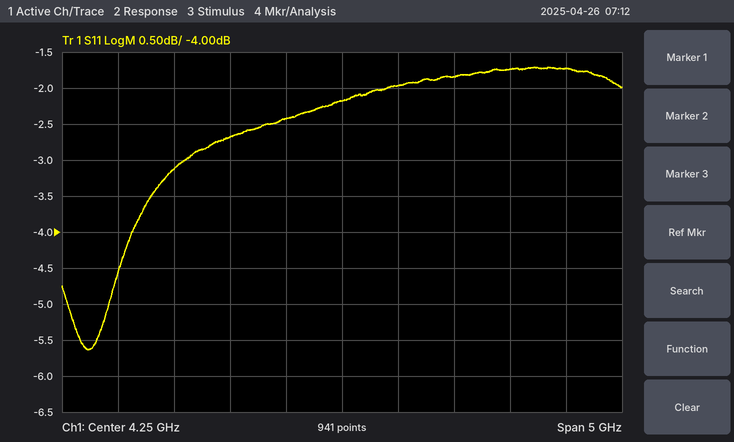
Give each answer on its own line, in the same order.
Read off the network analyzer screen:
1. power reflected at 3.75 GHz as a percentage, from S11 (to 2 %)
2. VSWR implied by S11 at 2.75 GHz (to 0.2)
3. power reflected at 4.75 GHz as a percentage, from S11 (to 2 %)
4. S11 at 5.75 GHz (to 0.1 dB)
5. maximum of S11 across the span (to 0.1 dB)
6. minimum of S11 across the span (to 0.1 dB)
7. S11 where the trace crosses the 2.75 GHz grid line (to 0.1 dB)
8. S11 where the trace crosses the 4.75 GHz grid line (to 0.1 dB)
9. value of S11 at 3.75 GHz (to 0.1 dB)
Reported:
58 %
5.6
64 %
-1.7 dB
-1.7 dB
-5.6 dB
-3.1 dB
-2.0 dB
-2.4 dB
